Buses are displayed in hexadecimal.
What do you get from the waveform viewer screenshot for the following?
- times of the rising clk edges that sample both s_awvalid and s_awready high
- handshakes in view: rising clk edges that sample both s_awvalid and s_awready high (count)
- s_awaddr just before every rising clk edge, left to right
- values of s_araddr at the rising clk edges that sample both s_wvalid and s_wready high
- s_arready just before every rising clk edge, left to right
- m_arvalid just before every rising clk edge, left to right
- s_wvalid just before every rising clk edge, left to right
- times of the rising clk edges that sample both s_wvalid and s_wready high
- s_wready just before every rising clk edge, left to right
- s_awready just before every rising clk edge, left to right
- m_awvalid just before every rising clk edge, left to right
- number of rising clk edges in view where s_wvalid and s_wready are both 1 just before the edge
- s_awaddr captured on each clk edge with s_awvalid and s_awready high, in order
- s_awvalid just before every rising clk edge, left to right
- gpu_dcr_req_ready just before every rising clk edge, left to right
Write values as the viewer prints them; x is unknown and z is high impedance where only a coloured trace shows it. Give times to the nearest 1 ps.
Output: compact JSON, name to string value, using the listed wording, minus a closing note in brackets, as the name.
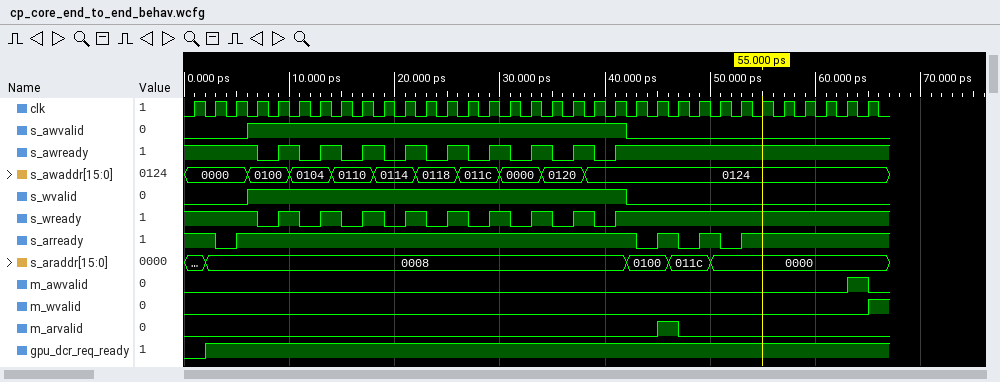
{"times of the rising clk edges that sample both s_awvalid and s_awready high": "7 ps, 11 ps, 15 ps, 19 ps, 23 ps, 27 ps, 31 ps, 35 ps, 39 ps", "handshakes in view: rising clk edges that sample both s_awvalid and s_awready high": "9", "s_awaddr just before every rising clk edge, left to right": "0000, 0000, 0000, 0100, 0100, 0104, 0104, 0110, 0110, 0114, 0114, 0118, 0118, 011c, 011c, 0000, 0000, 0120, 0120, 0124, 0124, 0124, 0124, 0124, 0124, 0124, 0124, 0124, 0124, 0124, 0124, 0124, 0124", "values of s_araddr at the rising clk edges that sample both s_wvalid and s_wready high": "0008, 0008, 0008, 0008, 0008, 0008, 0008, 0008, 0008", "s_arready just before every rising clk edge, left to right": "1 1 0 1 1 1 1 1 1 1 1 1 1 1 1 1 1 1 1 1 1 1 0 1 0 1 0 1 1 1 1 1 1", "m_arvalid just before every rising clk edge, left to right": "0 0 0 0 0 0 0 0 0 0 0 0 0 0 0 0 0 0 0 0 0 0 0 1 0 0 0 0 0 0 0 0 0", "s_wvalid just before every rising clk edge, left to right": "0 0 0 1 1 1 1 1 1 1 1 1 1 1 1 1 1 1 1 1 1 0 0 0 0 0 0 0 0 0 0 0 0", "times of the rising clk edges that sample both s_wvalid and s_wready high": "7 ps, 11 ps, 15 ps, 19 ps, 23 ps, 27 ps, 31 ps, 35 ps, 39 ps", "s_wready just before every rising clk edge, left to right": "1 1 1 1 0 1 0 1 0 1 0 1 0 1 0 1 0 1 0 1 0 1 1 1 1 1 1 1 1 1 1 1 1", "s_awready just before every rising clk edge, left to right": "1 1 1 1 0 1 0 1 0 1 0 1 0 1 0 1 0 1 0 1 0 1 1 1 1 1 1 1 1 1 1 1 1", "m_awvalid just before every rising clk edge, left to right": "0 0 0 0 0 0 0 0 0 0 0 0 0 0 0 0 0 0 0 0 0 0 0 0 0 0 0 0 0 0 0 0 1", "number of rising clk edges in view where s_wvalid and s_wready are both 1 just before the edge": "9", "s_awaddr captured on each clk edge with s_awvalid and s_awready high, in order": "0100, 0104, 0110, 0114, 0118, 011c, 0000, 0120, 0124", "s_awvalid just before every rising clk edge, left to right": "0 0 0 1 1 1 1 1 1 1 1 1 1 1 1 1 1 1 1 1 1 0 0 0 0 0 0 0 0 0 0 0 0", "gpu_dcr_req_ready just before every rising clk edge, left to right": "0 1 1 1 1 1 1 1 1 1 1 1 1 1 1 1 1 1 1 1 1 1 1 1 1 1 1 1 1 1 1 1 1"}
